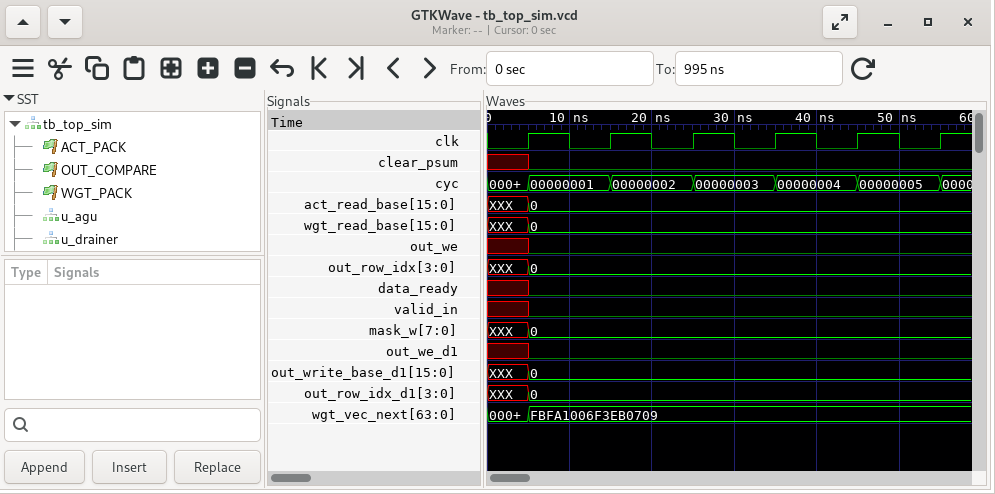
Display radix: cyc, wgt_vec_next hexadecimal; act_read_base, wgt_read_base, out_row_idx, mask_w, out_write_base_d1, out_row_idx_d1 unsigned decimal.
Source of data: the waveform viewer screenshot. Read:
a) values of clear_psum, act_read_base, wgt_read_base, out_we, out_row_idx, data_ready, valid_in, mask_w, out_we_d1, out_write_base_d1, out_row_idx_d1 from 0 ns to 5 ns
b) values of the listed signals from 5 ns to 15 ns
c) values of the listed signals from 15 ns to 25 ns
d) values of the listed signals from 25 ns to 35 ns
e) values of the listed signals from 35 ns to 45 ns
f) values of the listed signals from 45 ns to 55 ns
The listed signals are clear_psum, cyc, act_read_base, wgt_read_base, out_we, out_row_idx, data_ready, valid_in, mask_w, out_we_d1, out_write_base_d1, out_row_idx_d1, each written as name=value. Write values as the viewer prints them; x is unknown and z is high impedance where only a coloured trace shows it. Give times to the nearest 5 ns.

clear_psum=x, act_read_base=XXX, wgt_read_base=XXX, out_we=x, out_row_idx=XXX, data_ready=x, valid_in=x, mask_w=XXX, out_we_d1=x, out_write_base_d1=XXX, out_row_idx_d1=XXX
clear_psum=0, cyc=00000001, act_read_base=0, wgt_read_base=0, out_we=0, out_row_idx=0, data_ready=0, valid_in=0, mask_w=0, out_we_d1=0, out_write_base_d1=0, out_row_idx_d1=0
clear_psum=0, cyc=00000002, act_read_base=0, wgt_read_base=0, out_we=0, out_row_idx=0, data_ready=0, valid_in=0, mask_w=0, out_we_d1=0, out_write_base_d1=0, out_row_idx_d1=0
clear_psum=0, cyc=00000003, act_read_base=0, wgt_read_base=0, out_we=0, out_row_idx=0, data_ready=0, valid_in=0, mask_w=0, out_we_d1=0, out_write_base_d1=0, out_row_idx_d1=0
clear_psum=0, cyc=00000004, act_read_base=0, wgt_read_base=0, out_we=0, out_row_idx=0, data_ready=0, valid_in=0, mask_w=0, out_we_d1=0, out_write_base_d1=0, out_row_idx_d1=0
clear_psum=0, cyc=00000005, act_read_base=0, wgt_read_base=0, out_we=0, out_row_idx=0, data_ready=0, valid_in=0, mask_w=0, out_we_d1=0, out_write_base_d1=0, out_row_idx_d1=0
